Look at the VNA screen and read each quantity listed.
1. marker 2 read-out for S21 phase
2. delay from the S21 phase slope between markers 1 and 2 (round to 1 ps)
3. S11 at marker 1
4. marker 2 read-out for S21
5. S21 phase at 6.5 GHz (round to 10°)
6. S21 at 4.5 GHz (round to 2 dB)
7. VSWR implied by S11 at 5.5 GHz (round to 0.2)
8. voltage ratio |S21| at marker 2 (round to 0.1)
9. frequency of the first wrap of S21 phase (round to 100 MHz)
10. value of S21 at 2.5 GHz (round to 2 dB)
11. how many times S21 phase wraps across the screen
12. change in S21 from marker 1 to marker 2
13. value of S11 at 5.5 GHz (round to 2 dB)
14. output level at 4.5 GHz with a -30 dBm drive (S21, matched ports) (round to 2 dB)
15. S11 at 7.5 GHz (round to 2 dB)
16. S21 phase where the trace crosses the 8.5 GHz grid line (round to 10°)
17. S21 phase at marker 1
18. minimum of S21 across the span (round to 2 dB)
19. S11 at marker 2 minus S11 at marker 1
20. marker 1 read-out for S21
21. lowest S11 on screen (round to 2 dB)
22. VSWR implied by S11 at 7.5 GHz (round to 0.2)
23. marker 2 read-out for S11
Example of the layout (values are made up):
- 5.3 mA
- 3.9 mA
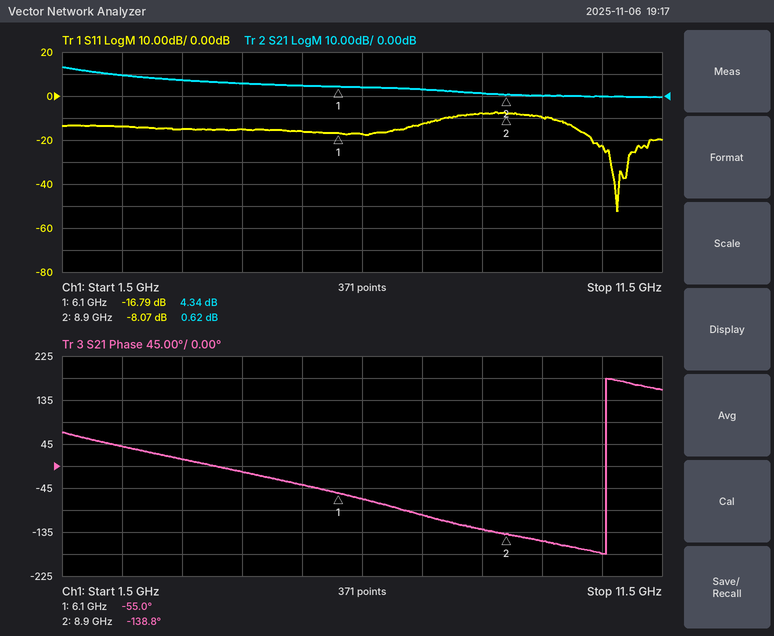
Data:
- -138.8°
- 83 ps
- -16.79 dB
- 0.62 dB
- -70°
- 6 dB
- 1.4
- 1.1
- 10.6 GHz
- 10 dB
- 1
- -3.72 dB
- -16 dB
- -24 dBm
- -12 dB
- -130°
- -55.0°
- 0 dB
- 8.72 dB
- 4.34 dB
- -52 dB
- 1.6
- -8.07 dB
